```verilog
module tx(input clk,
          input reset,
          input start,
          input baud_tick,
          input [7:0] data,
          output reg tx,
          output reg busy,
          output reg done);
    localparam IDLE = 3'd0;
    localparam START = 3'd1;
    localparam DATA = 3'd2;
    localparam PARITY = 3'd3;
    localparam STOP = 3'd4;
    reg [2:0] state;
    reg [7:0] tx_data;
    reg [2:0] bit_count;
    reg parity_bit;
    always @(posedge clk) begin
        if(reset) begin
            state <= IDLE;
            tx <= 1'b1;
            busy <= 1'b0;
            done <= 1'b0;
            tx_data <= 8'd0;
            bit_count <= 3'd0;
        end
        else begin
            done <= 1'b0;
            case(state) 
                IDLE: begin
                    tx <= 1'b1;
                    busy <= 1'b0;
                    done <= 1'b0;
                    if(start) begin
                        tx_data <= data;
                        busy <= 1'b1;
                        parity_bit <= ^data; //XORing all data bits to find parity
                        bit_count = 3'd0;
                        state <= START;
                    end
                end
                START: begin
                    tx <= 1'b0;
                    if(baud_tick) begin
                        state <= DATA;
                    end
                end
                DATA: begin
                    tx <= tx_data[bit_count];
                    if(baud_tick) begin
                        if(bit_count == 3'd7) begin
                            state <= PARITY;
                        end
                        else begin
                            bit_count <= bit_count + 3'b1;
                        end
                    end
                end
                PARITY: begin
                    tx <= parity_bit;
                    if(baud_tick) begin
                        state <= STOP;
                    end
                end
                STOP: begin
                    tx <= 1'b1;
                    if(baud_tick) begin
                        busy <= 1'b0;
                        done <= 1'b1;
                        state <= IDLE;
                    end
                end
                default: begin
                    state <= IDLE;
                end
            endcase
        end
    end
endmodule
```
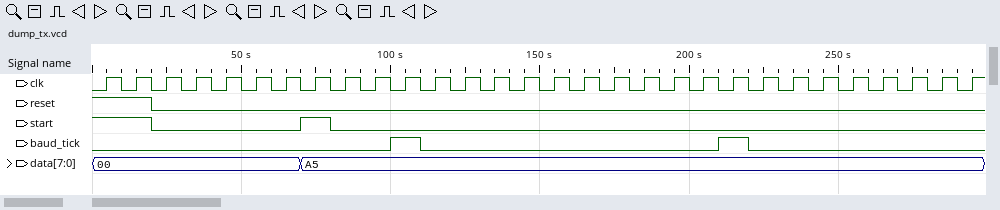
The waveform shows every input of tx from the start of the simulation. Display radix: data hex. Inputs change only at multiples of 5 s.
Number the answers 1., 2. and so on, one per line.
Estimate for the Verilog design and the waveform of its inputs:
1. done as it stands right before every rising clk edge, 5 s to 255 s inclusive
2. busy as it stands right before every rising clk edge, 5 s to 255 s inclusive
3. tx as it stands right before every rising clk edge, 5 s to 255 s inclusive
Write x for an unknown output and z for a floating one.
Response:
1. x 0 0 0 0 0 0 0 0 0 0 0 0 0 0 0 0 0 0 0 0 0 0 0 0 0
2. x 0 0 0 0 0 0 0 1 1 1 1 1 1 1 1 1 1 1 1 1 1 1 1 1 1
3. x 1 1 1 1 1 1 1 1 0 0 0 1 1 1 1 1 1 1 1 1 1 1 0 0 0
